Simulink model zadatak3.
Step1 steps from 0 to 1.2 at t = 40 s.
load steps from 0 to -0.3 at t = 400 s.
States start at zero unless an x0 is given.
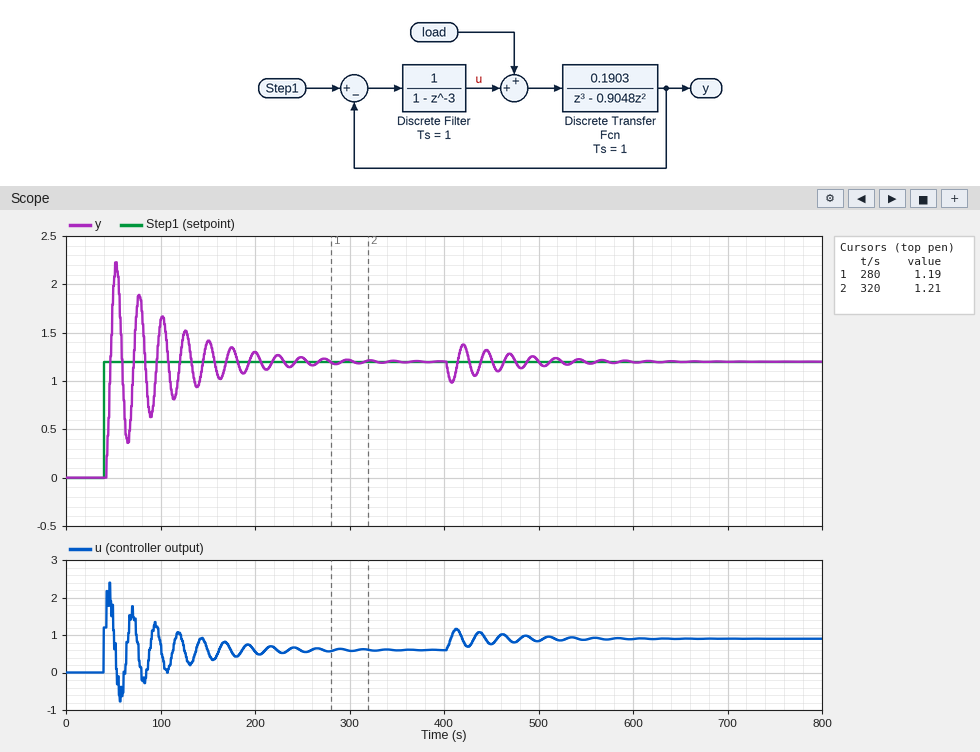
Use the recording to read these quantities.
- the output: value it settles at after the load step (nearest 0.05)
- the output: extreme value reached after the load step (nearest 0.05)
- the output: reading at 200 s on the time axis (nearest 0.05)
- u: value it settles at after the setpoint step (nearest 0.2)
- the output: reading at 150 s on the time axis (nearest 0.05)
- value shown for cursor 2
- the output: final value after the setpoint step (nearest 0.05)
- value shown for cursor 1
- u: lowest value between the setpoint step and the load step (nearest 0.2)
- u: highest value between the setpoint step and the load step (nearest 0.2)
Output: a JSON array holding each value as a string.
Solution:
["1.20", "1.00", "1.30", "0.6", "1.40", "1.21", "1.20", "1.19", "-0.8", "2.4"]
